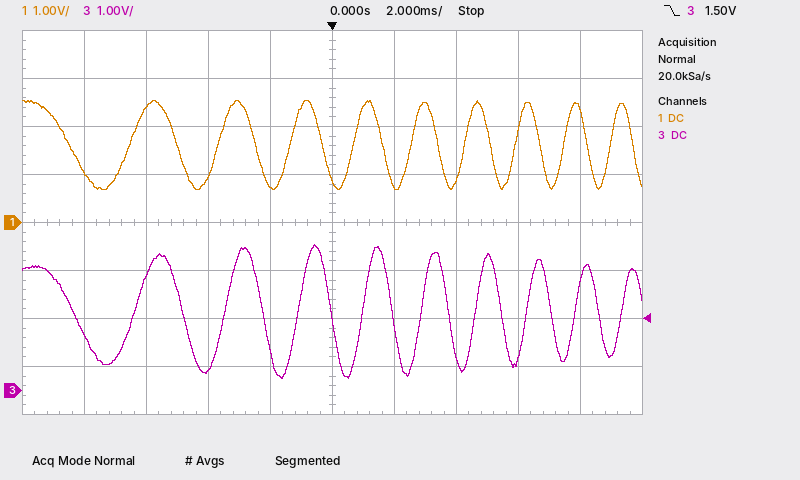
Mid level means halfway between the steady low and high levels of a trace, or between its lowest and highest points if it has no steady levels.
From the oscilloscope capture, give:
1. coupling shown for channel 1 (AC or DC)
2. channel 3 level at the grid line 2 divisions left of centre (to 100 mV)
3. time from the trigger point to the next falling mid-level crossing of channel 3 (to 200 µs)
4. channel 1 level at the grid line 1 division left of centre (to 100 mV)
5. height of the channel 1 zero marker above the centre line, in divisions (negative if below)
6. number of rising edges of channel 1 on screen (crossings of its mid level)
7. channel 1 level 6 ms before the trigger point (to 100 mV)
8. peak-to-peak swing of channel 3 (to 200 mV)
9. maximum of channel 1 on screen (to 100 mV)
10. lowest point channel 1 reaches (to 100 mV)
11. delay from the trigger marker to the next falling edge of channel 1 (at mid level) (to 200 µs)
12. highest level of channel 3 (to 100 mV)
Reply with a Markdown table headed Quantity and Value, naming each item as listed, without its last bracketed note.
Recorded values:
| Quantity | Value |
|---|---|
| coupling shown for channel 1 | DC |
| channel 3 level at the grid line 2 divisions left of centre | 400 mV |
| time from the trigger point to the next falling mid-level crossing of channel 3 | 2.0 ms |
| channel 1 level at the grid line 1 division left of centre | 800 mV |
| height of the channel 1 zero marker above the centre line, in divisions | 0.0 div |
| number of rising edges of channel 1 on screen | 9 |
| channel 1 level 6 ms before the trigger point | 2.4 V |
| peak-to-peak swing of channel 3 | 2.8 V |
| maximum of channel 1 on screen | 2.5 V |
| lowest point channel 1 reaches | 700 mV |
| delay from the trigger marker to the next falling edge of channel 1 (at mid level) | 1.6 ms |
| highest level of channel 3 | 3.0 V |
